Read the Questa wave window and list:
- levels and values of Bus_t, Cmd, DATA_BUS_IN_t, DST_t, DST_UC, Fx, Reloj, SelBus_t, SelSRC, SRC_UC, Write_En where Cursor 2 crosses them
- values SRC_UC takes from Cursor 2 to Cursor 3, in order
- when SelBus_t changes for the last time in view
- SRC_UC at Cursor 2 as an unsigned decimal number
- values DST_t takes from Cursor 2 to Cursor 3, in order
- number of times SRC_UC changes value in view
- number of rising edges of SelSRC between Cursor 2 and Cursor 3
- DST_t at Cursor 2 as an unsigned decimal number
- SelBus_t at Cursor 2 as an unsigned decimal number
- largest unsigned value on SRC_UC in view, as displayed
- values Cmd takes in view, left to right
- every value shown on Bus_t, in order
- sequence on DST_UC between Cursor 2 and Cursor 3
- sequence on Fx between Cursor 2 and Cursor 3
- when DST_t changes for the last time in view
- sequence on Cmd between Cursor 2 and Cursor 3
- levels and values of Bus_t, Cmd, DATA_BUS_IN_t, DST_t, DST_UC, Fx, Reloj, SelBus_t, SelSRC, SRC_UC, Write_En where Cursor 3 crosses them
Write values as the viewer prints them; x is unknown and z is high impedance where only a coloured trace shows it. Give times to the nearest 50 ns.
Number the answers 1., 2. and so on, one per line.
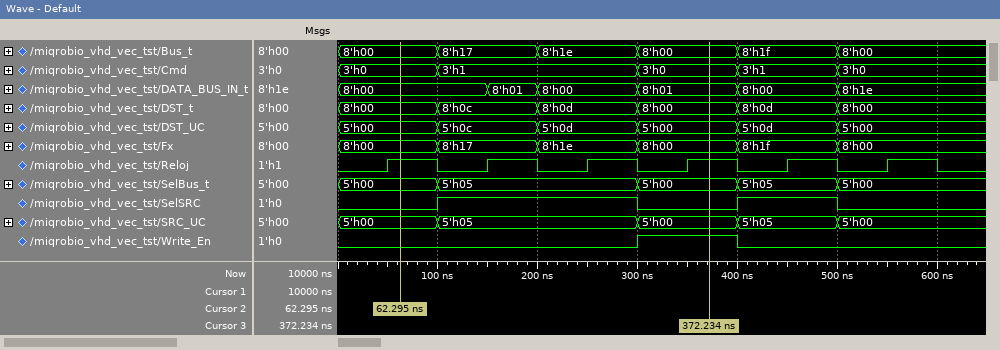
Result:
1. Bus_t=8'h00, Cmd=3'h0, DATA_BUS_IN_t=8'h00, DST_t=8'h00, DST_UC=5'h00, Fx=8'h00, Reloj=1, SelBus_t=5'h00, SelSRC=0, SRC_UC=5'h00, Write_En=0
2. 5'h00, 5'h05, 5'h00
3. 500 ns
4. 0
5. 8'h00, 8'h0c, 8'h0d, 8'h00
6. 4
7. 1
8. 0
9. 0
10. 5'h05
11. 3'h0, 3'h1, 3'h0, 3'h1, 3'h0
12. 8'h00, 8'h17, 8'h1e, 8'h00, 8'h1f, 8'h00
13. 5'h00, 5'h0c, 5'h0d, 5'h00
14. 8'h00, 8'h17, 8'h1e, 8'h00
15. 500 ns
16. 3'h0, 3'h1, 3'h0
17. Bus_t=8'h00, Cmd=3'h0, DATA_BUS_IN_t=8'h01, DST_t=8'h00, DST_UC=5'h00, Fx=8'h00, Reloj=1, SelBus_t=5'h00, SelSRC=0, SRC_UC=5'h00, Write_En=1
